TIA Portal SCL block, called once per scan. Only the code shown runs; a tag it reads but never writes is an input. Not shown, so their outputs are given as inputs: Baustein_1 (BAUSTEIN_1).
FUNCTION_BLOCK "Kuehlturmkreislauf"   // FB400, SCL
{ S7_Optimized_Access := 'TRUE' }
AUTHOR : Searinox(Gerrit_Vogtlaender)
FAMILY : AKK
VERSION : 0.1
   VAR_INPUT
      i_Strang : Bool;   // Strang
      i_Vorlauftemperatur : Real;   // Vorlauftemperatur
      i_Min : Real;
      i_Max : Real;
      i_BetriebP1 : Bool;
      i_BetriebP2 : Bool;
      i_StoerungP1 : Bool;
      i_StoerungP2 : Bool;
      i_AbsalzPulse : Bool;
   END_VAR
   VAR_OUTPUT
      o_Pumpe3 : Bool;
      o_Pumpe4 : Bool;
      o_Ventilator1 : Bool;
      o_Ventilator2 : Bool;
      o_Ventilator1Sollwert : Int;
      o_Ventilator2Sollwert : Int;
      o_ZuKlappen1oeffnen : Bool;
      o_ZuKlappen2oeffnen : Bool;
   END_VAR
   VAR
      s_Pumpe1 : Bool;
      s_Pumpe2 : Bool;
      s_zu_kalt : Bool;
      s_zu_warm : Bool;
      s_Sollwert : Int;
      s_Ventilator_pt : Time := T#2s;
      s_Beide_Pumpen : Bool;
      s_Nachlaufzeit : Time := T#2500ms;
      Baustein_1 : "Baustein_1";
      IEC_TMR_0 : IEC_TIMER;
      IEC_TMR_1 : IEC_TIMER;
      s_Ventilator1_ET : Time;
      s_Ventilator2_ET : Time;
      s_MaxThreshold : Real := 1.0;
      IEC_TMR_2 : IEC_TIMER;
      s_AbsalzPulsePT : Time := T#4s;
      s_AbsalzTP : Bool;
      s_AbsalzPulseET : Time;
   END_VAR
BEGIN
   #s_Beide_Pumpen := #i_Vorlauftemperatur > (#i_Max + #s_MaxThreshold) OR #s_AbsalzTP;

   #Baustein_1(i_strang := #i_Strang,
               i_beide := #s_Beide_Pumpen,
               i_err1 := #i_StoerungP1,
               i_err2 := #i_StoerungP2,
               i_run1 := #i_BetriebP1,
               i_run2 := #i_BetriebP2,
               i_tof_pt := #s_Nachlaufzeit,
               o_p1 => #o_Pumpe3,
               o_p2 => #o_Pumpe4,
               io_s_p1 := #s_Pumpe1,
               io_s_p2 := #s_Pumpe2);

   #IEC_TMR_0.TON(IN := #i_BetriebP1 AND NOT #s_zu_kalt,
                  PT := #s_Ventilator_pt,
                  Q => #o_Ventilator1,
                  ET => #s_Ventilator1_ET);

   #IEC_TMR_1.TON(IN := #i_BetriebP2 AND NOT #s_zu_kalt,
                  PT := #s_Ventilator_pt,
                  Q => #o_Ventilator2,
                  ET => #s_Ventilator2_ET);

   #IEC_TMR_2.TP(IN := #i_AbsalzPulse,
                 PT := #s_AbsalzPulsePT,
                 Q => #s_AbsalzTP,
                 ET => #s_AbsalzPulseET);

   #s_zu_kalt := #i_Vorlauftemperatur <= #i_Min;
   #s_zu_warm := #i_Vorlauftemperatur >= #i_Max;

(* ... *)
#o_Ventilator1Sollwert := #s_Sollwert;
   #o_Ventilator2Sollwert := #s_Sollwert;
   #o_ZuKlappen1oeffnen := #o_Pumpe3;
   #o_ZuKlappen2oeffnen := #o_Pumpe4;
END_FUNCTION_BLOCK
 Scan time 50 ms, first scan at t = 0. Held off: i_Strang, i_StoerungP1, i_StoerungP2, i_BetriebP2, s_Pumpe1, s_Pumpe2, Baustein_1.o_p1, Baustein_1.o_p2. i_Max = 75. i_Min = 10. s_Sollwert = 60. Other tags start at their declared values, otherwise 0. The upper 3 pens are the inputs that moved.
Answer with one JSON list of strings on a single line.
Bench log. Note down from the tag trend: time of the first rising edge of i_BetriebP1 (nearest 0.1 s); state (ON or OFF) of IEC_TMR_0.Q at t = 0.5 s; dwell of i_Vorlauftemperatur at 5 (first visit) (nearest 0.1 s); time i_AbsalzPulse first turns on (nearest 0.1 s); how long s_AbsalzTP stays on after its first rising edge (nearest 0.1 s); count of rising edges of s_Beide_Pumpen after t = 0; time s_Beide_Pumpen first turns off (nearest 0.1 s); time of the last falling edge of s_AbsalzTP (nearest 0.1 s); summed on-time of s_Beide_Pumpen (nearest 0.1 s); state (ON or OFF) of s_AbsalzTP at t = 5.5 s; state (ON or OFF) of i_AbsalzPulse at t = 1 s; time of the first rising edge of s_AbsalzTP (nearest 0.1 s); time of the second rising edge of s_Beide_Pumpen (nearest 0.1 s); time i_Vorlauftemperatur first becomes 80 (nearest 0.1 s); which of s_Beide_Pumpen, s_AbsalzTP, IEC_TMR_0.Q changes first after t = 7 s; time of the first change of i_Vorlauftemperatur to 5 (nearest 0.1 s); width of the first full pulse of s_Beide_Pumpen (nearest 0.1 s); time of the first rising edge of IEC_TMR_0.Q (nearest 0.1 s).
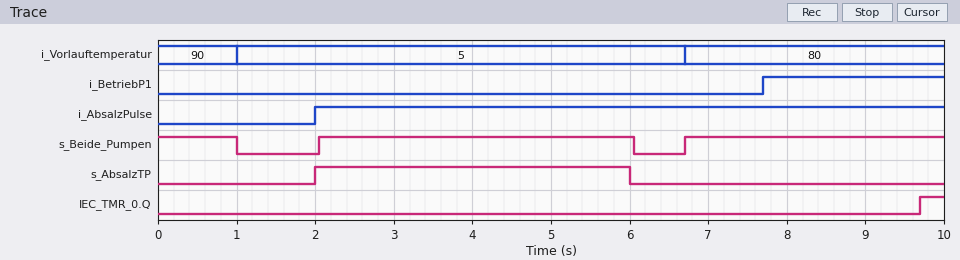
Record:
["7.7 s", "OFF", "5.7 s", "2.0 s", "4.0 s", "2", "1.0 s", "6.0 s", "8.3 s", "ON", "OFF", "2.0 s", "6.7 s", "6.7 s", "IEC_TMR_0.Q", "1.0 s", "4.0 s", "9.7 s"]
